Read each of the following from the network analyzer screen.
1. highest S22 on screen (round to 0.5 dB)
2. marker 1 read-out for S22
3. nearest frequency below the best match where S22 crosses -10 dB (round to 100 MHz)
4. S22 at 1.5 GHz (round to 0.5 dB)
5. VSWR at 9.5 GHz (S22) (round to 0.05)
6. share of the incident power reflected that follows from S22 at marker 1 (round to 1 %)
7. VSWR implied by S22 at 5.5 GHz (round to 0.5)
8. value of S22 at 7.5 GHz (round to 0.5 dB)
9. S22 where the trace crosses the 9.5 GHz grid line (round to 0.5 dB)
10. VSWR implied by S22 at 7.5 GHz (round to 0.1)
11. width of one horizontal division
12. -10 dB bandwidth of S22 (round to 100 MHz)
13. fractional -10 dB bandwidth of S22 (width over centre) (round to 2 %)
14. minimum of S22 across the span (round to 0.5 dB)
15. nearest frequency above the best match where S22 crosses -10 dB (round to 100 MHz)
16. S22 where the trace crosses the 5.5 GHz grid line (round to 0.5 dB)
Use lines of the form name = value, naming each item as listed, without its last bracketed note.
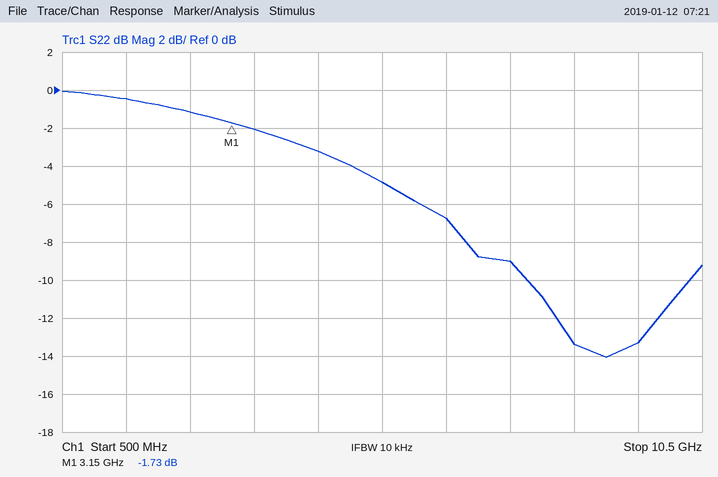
highest S22 on screen = 0.0 dB
marker 1 read-out for S22 = -1.73 dB
nearest frequency below the best match where S22 crosses -10 dB = 7.8 GHz
S22 at 1.5 GHz = -0.5 dB
VSWR at 9.5 GHz (S22) = 1.55
share of the incident power reflected that follows from S22 at marker 1 = 67 %
VSWR implied by S22 at 5.5 GHz = 3.5
value of S22 at 7.5 GHz = -9.0 dB
S22 where the trace crosses the 9.5 GHz grid line = -13.5 dB
VSWR implied by S22 at 7.5 GHz = 2.1
width of one horizontal division = 1 GHz
-10 dB bandwidth of S22 = 2.5 GHz
fractional -10 dB bandwidth of S22 (width over centre) = 28 %
minimum of S22 across the span = -14.0 dB
nearest frequency above the best match where S22 crosses -10 dB = 10.3 GHz
S22 where the trace crosses the 5.5 GHz grid line = -5.0 dB
